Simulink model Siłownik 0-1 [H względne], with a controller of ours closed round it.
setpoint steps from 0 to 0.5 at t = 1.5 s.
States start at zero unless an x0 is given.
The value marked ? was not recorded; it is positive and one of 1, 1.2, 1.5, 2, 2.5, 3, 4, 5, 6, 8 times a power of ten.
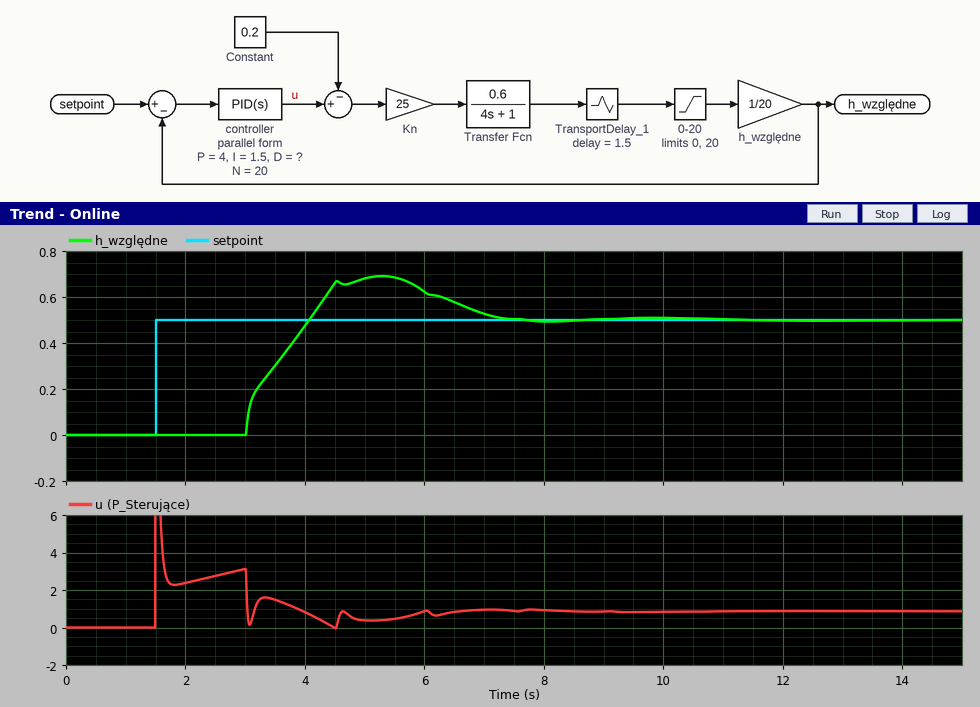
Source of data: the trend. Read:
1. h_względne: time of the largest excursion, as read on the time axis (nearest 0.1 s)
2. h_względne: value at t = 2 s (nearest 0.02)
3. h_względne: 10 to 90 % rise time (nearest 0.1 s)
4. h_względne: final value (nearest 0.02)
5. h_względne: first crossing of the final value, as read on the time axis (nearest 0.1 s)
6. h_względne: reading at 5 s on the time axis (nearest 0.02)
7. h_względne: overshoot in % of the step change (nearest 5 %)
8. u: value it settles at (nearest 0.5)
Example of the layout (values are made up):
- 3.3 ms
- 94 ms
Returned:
- 5.3 s
- 0.00
- 0.9 s
- 0.50
- 4.1 s
- 0.68
- 40 %
- 1.0
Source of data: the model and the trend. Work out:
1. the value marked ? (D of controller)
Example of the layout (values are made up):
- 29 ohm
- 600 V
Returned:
- 2
